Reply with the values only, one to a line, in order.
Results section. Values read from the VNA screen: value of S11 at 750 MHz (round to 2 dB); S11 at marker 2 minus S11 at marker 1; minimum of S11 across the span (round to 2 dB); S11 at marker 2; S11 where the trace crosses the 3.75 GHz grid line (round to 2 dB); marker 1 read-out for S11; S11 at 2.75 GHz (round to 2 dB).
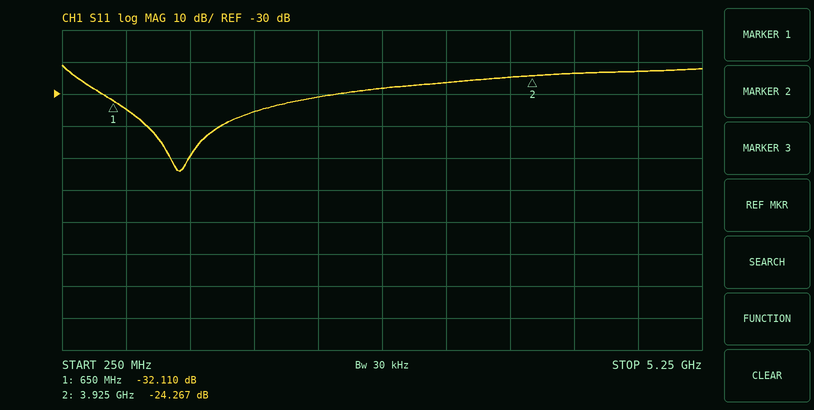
-34 dB
7.843 dB
-54 dB
-24.267 dB
-24 dB
-32.110 dB
-28 dB
